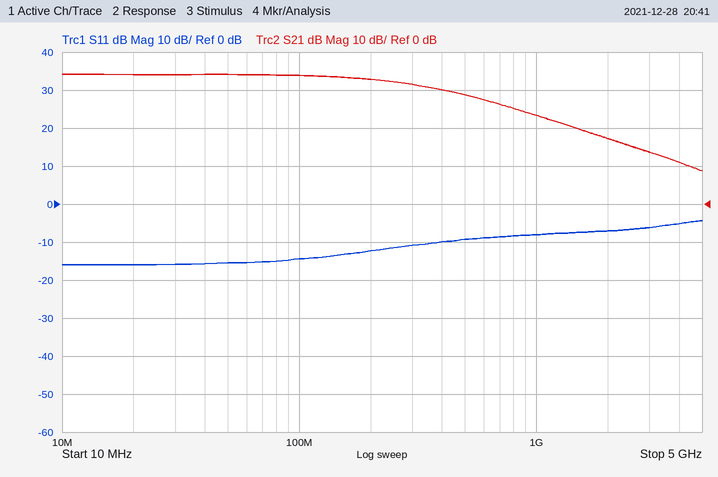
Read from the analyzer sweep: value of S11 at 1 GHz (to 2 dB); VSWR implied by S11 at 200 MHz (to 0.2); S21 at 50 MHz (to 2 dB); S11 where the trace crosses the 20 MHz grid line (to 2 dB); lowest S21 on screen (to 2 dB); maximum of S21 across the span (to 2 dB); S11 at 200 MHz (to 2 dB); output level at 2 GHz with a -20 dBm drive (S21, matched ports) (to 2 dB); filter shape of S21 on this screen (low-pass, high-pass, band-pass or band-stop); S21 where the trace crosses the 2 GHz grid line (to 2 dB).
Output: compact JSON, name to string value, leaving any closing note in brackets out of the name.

{"value of S11 at 1 GHz": "-8 dB", "VSWR implied by S11 at 200 MHz": "1.6", "S21 at 50 MHz": "34 dB", "S11 where the trace crosses the 20 MHz grid line": "-16 dB", "lowest S21 on screen": "8 dB", "maximum of S21 across the span": "34 dB", "S11 at 200 MHz": "-12 dB", "output level at 2 GHz with a -20 dBm drive (S21, matched ports)": "-2 dBm", "filter shape of S21 on this screen": "low-pass", "S21 where the trace crosses the 2 GHz grid line": "18 dB"}
